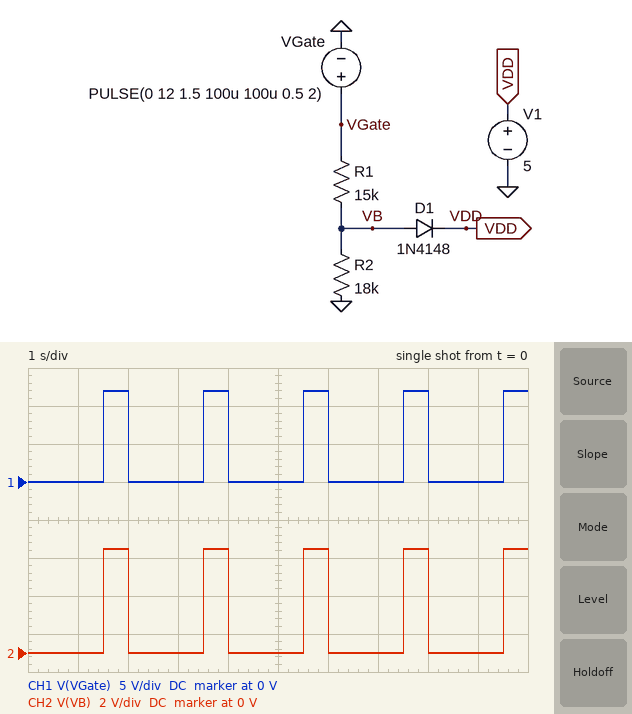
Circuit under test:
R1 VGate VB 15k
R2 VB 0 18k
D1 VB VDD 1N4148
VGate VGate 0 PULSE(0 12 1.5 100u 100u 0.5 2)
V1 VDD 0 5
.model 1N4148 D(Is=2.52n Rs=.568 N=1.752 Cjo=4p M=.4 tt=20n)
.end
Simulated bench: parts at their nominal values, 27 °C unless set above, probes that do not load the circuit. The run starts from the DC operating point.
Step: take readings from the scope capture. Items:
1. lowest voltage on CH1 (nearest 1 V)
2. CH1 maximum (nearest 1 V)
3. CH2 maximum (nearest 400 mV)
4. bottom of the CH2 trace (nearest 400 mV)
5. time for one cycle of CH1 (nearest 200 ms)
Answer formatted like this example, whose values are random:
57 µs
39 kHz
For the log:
0 V
12 V
5.6 V
0 V
2.0 s
